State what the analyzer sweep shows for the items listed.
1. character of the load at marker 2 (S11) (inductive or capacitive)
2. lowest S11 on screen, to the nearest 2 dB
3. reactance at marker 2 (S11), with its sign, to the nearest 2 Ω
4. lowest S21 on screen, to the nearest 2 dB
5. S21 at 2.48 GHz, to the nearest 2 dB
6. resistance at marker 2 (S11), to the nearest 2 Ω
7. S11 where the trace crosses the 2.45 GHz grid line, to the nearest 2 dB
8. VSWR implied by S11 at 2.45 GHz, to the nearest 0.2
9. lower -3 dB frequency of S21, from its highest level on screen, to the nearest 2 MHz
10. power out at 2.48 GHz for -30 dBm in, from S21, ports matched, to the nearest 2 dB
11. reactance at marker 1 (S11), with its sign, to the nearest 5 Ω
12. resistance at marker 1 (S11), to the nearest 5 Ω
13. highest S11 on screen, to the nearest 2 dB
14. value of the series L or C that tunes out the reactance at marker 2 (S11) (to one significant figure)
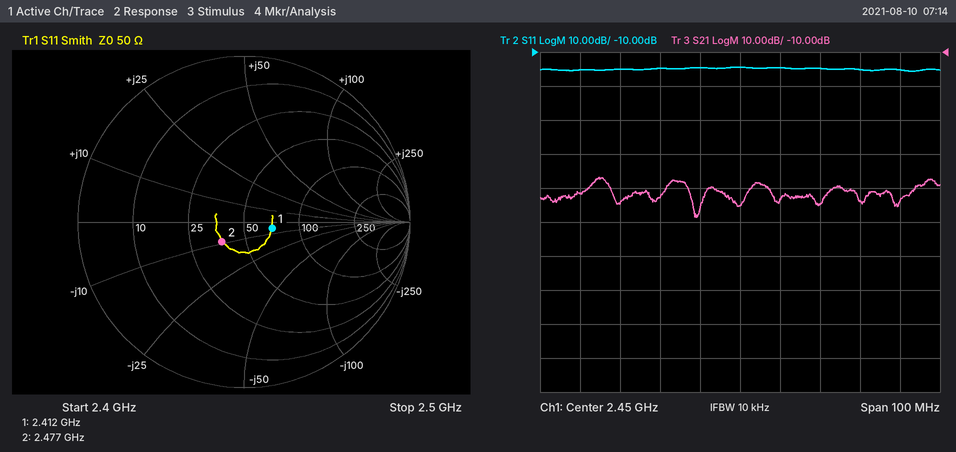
capacitive
-16 dB
-10 Ω
-58 dB
-54 dB
38 Ω
-14 dB
1.4
2.412 GHz
-84 dBm
-5 Ω
70 Ω
-14 dB
600 pH
